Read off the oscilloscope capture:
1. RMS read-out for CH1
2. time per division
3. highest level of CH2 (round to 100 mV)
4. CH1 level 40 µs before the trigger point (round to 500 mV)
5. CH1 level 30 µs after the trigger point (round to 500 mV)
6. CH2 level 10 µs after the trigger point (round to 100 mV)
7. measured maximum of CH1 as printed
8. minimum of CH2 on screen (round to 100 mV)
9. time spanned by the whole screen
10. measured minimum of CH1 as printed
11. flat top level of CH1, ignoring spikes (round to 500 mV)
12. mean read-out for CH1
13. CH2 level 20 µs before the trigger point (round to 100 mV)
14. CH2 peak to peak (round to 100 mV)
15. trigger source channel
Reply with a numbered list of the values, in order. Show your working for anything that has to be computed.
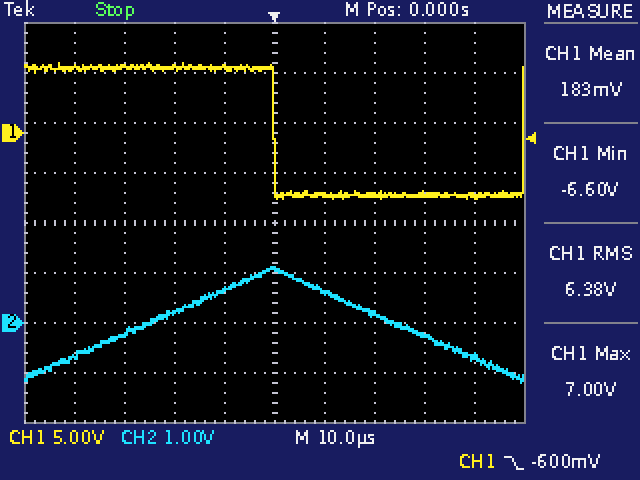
1. 6.38 V
2. 10 µs
3. 1.1 V
4. 6.5 V
5. -6.0 V
6. 600 mV
7. 7.00 V
8. -1.2 V
9. 100 µs
10. -6.60 V
11. 6.5 V
12. 183 mV
13. 200 mV
14. 1.1 V − (-1.2 V) = 2.3 V
15. CH1
